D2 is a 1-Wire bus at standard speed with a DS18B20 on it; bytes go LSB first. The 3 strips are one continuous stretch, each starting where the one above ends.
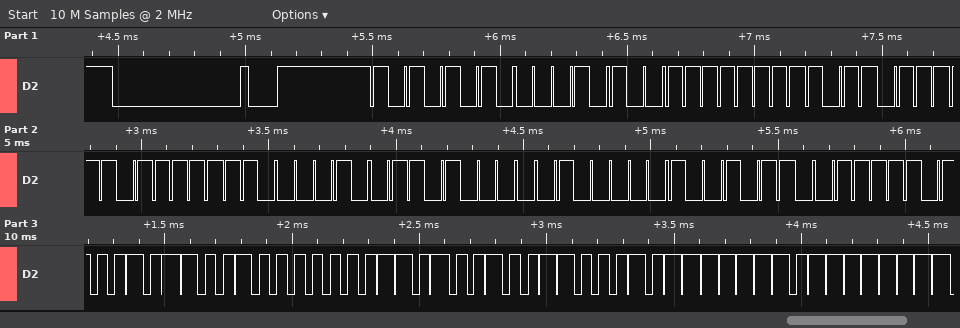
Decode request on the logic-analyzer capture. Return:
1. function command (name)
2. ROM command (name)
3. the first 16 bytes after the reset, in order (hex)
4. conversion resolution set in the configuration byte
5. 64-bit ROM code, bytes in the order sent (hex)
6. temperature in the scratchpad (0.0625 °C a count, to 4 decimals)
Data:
Read Scratchpad
Match ROM
55 28 FF ED FB 43 16 04 69 BE 34 01 4B 46 7F FF
12 bits
28 FF ED FB 43 16 04 69
19.2500 °C
